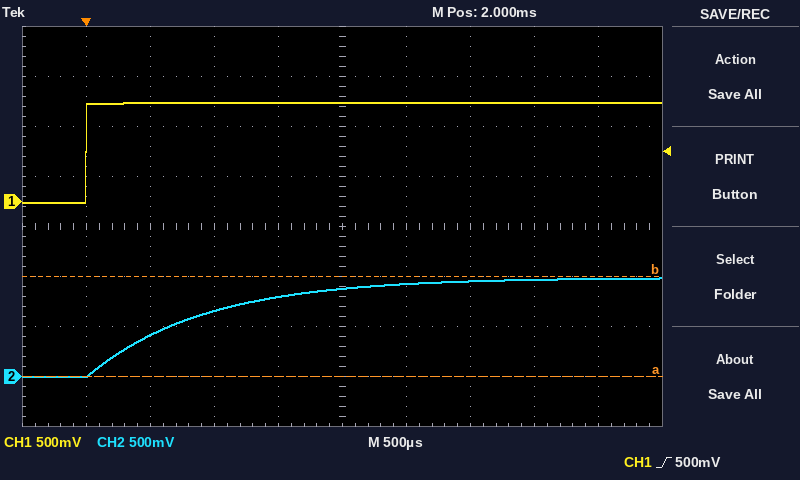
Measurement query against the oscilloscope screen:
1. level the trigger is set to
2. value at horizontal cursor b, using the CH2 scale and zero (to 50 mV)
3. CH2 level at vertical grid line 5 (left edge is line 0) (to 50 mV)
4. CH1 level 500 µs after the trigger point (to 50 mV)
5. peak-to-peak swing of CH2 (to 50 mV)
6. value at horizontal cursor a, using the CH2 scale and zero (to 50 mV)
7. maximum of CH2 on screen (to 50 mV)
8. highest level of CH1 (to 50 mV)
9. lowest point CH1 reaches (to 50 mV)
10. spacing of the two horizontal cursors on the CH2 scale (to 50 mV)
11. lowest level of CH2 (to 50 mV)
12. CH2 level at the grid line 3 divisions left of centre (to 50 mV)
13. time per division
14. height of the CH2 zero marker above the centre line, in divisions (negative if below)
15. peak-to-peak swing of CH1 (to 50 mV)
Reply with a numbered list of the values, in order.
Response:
1. 500 mV
2. 1.00 V
3. 900 mV
4. 1.00 V
5. 1.00 V
6. 0 mV
7. 1.00 V
8. 1.00 V
9. 0 mV
10. 1.00 V
11. 0 mV
12. 400 mV
13. 500 µs
14. -3.0 div
15. 1.00 V
